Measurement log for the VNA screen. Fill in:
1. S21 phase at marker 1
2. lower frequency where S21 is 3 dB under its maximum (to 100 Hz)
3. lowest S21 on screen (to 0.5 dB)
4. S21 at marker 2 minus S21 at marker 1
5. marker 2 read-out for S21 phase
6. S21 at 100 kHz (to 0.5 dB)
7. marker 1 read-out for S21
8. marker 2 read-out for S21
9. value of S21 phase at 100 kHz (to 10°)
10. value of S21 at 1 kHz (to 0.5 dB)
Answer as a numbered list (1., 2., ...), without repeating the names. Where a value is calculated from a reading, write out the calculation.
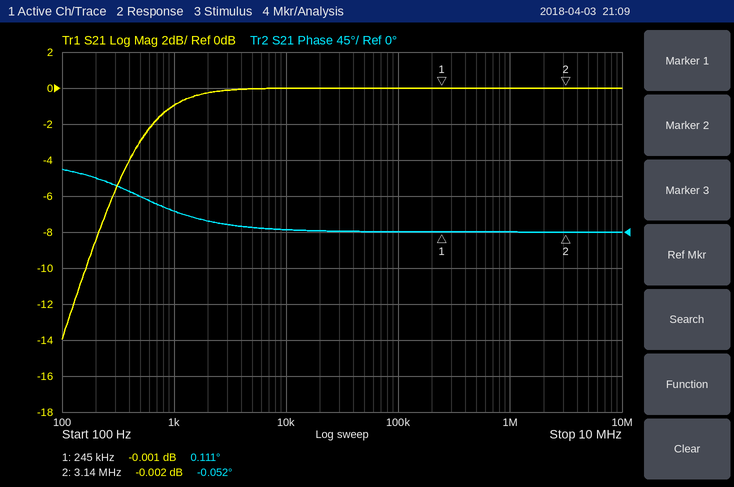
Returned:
1. 0.111°
2. 500 Hz
3. -14.0 dB
4. -0.002 − (-0.001) = -0.001 dB
5. -0.052°
6. 0.0 dB
7. -0.001 dB
8. -0.002 dB
9. 0°
10. -1.0 dB
